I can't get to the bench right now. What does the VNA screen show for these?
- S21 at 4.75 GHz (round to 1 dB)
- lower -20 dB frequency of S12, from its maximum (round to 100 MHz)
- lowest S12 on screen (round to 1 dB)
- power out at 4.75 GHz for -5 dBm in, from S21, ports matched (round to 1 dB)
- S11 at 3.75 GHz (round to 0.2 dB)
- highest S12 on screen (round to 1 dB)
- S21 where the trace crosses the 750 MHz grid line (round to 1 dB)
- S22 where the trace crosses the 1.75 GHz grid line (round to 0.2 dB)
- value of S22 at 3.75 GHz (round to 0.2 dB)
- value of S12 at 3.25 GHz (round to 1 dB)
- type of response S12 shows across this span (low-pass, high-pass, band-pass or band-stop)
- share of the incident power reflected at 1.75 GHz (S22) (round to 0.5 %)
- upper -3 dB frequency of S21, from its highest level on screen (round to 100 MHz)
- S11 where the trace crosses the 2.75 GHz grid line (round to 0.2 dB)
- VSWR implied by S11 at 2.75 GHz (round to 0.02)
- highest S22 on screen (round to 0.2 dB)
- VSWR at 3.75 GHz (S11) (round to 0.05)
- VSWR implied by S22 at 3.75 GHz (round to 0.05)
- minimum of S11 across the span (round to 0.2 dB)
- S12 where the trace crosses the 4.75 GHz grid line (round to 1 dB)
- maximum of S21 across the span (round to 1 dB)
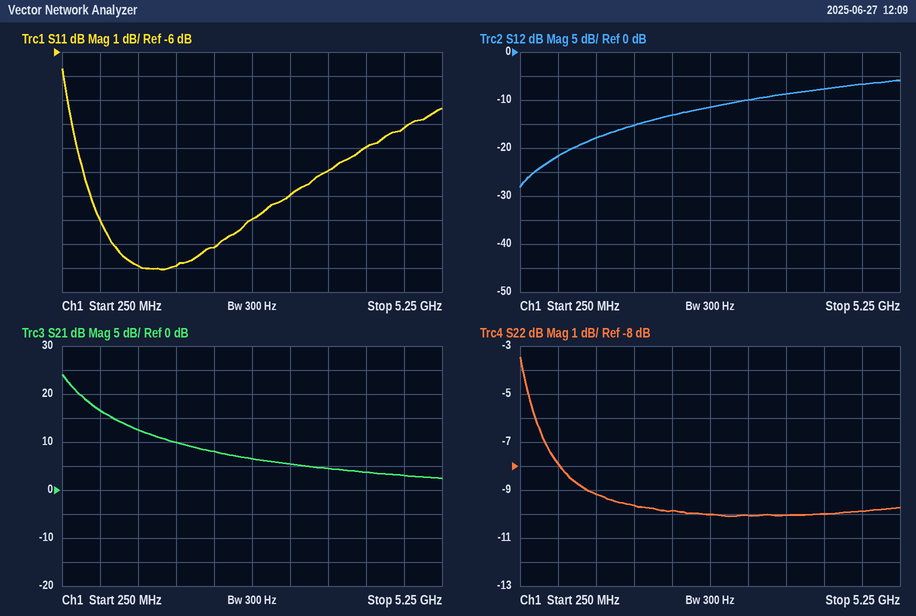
3 dB
400 MHz
-28 dB
-2 dBm
-11.0 dB
-6 dB
17 dB
-9.6 dB
-10.0 dB
-10 dB
high-pass
11.0 %
400 MHz
-13.0 dB
1.58
-3.4 dB
1.80
1.90
-15.0 dB
-7 dB
24 dB
